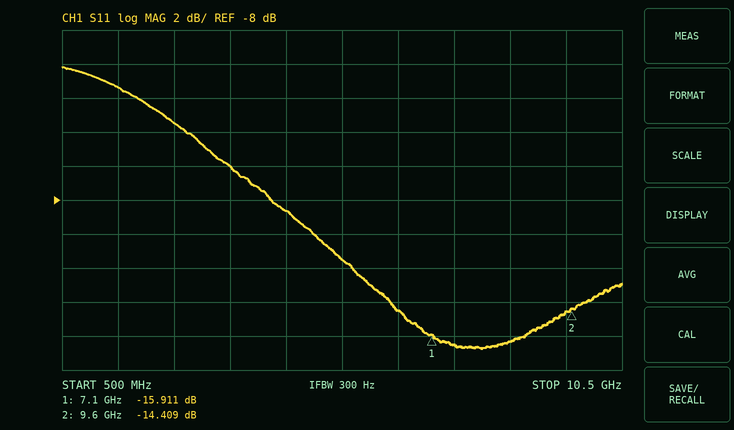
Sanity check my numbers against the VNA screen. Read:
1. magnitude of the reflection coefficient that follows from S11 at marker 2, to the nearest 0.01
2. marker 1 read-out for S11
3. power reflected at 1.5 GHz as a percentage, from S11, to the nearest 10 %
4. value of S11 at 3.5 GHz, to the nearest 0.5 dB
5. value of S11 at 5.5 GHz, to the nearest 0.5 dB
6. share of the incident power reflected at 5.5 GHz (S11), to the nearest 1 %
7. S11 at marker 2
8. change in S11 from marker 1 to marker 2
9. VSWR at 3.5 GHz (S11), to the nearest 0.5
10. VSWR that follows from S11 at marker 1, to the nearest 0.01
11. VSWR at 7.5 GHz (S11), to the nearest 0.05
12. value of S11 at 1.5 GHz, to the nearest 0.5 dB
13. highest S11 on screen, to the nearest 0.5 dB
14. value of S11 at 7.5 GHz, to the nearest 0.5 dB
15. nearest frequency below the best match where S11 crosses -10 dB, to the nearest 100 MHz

0.19
-15.911 dB
70 %
-6.0 dB
-11.5 dB
7 %
-14.409 dB
1.502 dB
3.0
1.38
1.35
-1.5 dB
0.0 dB
-16.5 dB
5.0 GHz
